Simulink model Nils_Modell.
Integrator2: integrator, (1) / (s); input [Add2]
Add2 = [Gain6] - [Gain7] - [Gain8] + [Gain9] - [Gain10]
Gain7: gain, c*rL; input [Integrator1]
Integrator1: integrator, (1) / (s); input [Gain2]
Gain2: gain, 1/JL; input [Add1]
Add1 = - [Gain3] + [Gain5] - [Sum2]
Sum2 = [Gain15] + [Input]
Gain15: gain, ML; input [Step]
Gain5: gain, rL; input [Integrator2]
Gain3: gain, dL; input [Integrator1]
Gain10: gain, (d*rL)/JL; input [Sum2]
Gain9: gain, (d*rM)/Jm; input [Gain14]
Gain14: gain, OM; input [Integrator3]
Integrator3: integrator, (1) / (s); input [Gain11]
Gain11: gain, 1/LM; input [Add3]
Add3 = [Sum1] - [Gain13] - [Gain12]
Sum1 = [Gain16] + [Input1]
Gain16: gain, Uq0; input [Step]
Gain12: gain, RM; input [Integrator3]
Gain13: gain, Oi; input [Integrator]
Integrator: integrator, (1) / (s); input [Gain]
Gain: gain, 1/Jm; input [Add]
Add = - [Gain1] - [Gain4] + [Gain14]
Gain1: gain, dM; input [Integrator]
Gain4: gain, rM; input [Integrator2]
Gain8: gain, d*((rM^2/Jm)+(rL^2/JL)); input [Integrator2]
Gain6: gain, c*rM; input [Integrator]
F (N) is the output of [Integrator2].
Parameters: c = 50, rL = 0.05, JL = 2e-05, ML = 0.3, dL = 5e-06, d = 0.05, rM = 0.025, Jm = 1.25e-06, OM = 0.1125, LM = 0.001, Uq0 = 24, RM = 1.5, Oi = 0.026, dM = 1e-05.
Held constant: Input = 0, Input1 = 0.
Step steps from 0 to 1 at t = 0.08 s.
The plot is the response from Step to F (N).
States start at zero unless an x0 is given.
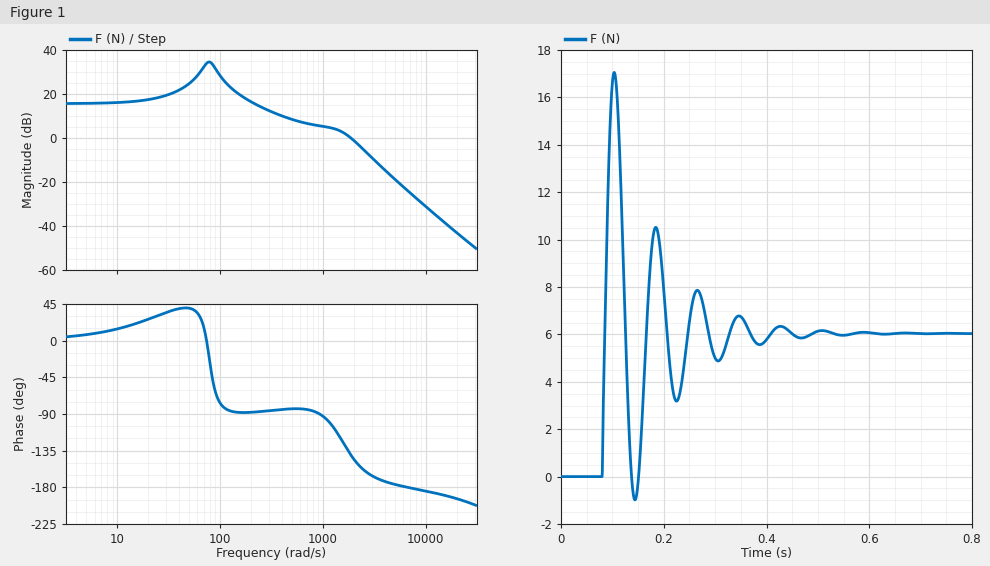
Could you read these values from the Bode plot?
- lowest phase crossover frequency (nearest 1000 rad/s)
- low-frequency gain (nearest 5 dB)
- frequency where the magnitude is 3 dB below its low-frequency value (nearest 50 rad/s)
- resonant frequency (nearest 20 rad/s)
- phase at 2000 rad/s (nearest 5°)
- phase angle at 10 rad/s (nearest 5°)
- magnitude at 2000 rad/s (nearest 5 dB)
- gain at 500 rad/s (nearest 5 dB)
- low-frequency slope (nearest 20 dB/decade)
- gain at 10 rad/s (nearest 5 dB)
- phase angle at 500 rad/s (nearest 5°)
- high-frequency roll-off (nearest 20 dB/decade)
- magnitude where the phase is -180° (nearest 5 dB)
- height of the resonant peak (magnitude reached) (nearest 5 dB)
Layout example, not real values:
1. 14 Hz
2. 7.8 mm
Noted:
1. 7000 rad/s
2. 15 dB
3. 300 rad/s
4. 80 rad/s
5. -145°
6. 15°
7. 0 dB
8. 10 dB
9. 0 dB/decade
10. 15 dB
11. -85°
12. -40 dB/decade
13. -25 dB
14. 35 dB
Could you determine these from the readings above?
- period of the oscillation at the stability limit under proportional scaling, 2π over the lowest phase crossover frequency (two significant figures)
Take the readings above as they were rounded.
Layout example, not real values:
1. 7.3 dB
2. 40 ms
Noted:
1. 0.00090 s
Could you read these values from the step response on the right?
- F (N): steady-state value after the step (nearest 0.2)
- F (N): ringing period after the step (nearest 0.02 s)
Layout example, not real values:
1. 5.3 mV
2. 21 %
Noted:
1. 6.0
2. 0.08 s
